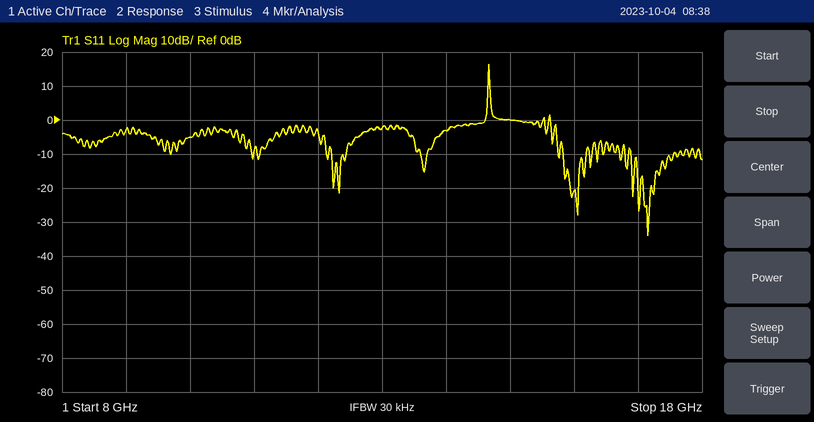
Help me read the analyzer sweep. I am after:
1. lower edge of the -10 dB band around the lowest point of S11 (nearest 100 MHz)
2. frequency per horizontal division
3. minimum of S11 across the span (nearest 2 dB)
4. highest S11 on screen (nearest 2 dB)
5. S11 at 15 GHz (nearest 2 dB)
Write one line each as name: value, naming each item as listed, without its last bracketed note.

lower edge of the -10 dB band around the lowest point of S11: 16.9 GHz
frequency per horizontal division: 1 GHz
minimum of S11 across the span: -34 dB
highest S11 on screen: 16 dB
S11 at 15 GHz: 0 dB
